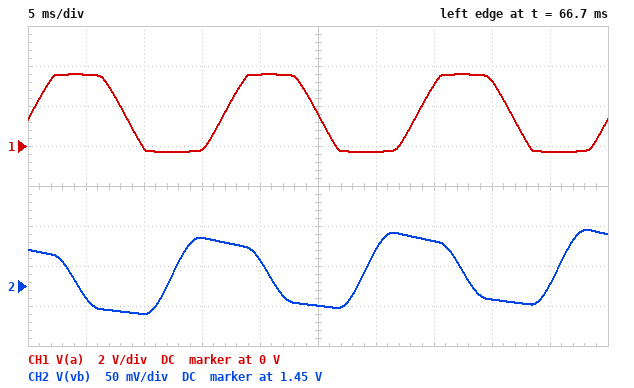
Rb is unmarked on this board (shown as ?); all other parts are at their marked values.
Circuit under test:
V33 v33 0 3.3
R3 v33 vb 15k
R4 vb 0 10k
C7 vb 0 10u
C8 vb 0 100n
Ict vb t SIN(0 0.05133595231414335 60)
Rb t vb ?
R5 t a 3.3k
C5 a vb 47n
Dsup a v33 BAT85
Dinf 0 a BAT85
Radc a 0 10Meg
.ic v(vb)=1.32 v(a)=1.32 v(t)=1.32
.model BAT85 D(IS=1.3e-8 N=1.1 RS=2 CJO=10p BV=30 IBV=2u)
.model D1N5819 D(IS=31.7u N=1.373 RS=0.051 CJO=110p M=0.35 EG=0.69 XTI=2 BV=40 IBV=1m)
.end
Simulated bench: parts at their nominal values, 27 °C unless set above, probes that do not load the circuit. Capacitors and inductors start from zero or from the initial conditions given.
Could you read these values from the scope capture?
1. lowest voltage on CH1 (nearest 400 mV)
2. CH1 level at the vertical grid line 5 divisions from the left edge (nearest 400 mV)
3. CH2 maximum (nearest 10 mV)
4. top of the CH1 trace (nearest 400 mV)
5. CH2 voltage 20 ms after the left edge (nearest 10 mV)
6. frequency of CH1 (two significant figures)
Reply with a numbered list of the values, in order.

1. -400 mV
2. 1.6 V
3. 1.52 V
4. 3.6 V
5. 1.48 V
6. 60 Hz
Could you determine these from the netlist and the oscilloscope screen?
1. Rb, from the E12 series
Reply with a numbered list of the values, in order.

1. 56 Ω
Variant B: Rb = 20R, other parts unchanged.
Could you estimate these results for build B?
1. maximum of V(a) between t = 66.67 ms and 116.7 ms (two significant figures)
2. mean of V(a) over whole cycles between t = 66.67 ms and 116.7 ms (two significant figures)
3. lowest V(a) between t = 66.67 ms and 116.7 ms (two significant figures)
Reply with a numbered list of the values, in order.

1. 2.3 V
2. 1.3 V
3. 290 mV
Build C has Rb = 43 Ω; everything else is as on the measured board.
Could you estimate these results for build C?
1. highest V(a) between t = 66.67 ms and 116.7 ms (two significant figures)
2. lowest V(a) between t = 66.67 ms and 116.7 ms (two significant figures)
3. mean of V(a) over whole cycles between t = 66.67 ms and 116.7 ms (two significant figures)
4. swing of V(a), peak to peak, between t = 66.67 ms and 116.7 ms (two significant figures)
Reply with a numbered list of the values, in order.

1. 3.5 V
2. -270 mV
3. 1.5 V
4. 3.8 V
